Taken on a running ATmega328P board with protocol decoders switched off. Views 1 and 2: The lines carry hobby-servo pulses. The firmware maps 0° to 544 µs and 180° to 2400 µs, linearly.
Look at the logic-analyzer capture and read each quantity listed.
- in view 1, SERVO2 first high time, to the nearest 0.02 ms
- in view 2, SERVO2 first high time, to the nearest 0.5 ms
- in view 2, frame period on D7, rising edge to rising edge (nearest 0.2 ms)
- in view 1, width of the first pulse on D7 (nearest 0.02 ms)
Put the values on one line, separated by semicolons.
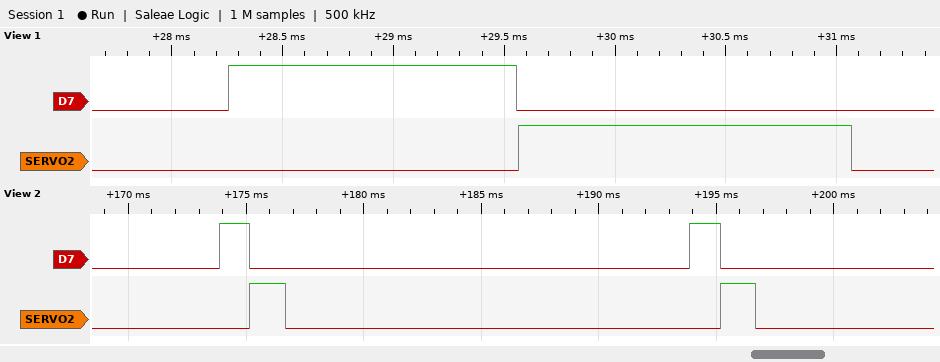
1.50 ms; 1.5 ms; 20.0 ms; 1.30 ms
